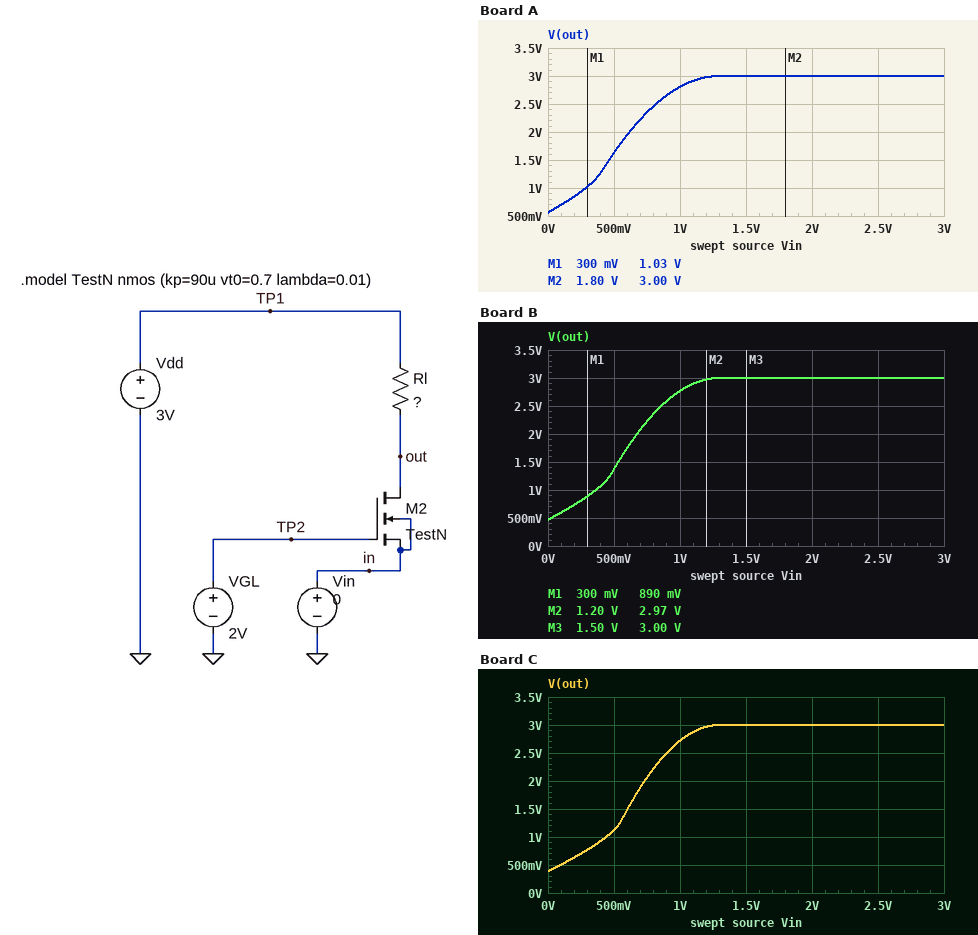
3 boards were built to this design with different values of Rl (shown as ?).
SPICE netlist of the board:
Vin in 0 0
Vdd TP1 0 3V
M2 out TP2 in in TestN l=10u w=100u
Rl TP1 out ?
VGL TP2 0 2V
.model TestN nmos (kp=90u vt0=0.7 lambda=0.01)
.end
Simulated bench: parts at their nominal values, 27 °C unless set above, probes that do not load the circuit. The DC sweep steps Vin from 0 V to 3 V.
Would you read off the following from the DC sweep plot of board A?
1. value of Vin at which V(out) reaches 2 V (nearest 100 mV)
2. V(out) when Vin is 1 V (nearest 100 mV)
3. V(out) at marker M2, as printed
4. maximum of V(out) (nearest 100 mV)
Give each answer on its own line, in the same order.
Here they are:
600 mV
2.8 V
3.00 V
3.0 V
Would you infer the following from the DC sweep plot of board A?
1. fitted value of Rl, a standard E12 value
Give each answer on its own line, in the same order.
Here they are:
4.7 kΩ
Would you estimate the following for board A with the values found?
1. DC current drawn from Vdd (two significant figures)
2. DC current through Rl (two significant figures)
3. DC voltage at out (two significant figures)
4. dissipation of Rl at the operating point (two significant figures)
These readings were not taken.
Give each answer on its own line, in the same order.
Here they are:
520 µA
520 µA
560 mV
1.3 mW
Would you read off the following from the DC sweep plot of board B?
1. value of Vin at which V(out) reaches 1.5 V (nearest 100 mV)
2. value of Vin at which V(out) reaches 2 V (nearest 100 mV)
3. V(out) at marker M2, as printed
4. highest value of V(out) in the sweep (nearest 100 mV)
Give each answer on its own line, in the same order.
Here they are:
500 mV
700 mV
2.97 V
3.0 V
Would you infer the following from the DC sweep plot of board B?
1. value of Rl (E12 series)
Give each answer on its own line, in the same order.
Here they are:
5.6 kΩ
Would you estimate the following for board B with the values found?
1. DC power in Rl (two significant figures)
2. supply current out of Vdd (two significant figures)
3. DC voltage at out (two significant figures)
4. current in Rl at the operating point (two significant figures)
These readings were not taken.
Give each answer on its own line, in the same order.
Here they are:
1.1 mW
450 µA
470 mV
450 µA
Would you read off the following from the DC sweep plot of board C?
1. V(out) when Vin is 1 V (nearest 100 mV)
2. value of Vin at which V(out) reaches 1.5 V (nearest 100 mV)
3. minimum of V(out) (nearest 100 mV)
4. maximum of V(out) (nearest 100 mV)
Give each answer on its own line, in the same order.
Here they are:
2.7 V
600 mV
400 mV
3.0 V
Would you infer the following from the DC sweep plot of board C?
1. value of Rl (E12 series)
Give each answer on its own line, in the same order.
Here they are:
6.8 kΩ
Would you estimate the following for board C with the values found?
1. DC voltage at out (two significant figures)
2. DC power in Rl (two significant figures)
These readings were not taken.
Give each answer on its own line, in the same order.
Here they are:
380 mV
1.0 mW
